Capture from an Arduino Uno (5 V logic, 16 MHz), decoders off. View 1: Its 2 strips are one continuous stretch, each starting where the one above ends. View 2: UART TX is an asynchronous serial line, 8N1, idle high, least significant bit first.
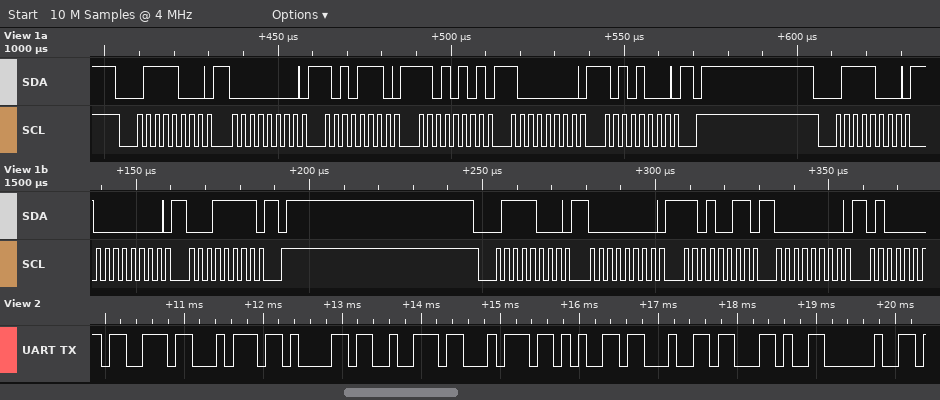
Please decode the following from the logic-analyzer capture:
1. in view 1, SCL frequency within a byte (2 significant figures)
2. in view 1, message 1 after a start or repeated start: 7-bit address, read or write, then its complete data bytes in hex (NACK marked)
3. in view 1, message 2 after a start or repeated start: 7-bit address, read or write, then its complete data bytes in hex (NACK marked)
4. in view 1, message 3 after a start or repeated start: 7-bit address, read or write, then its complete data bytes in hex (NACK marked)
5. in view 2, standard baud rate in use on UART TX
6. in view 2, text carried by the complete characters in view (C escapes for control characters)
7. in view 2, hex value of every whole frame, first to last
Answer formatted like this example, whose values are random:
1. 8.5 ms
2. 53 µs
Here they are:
1. 400 kHz
2. 0x3C write: 00 AE D5 80 A8
3. 0x3C write: 00 1F
4. 0x3C write: 00 D3 00
5. 9600 baud
6. "started, "
7. 0x73 0x74 0x61 0x72 0x74 0x65 0x64 0x2C 0x20
